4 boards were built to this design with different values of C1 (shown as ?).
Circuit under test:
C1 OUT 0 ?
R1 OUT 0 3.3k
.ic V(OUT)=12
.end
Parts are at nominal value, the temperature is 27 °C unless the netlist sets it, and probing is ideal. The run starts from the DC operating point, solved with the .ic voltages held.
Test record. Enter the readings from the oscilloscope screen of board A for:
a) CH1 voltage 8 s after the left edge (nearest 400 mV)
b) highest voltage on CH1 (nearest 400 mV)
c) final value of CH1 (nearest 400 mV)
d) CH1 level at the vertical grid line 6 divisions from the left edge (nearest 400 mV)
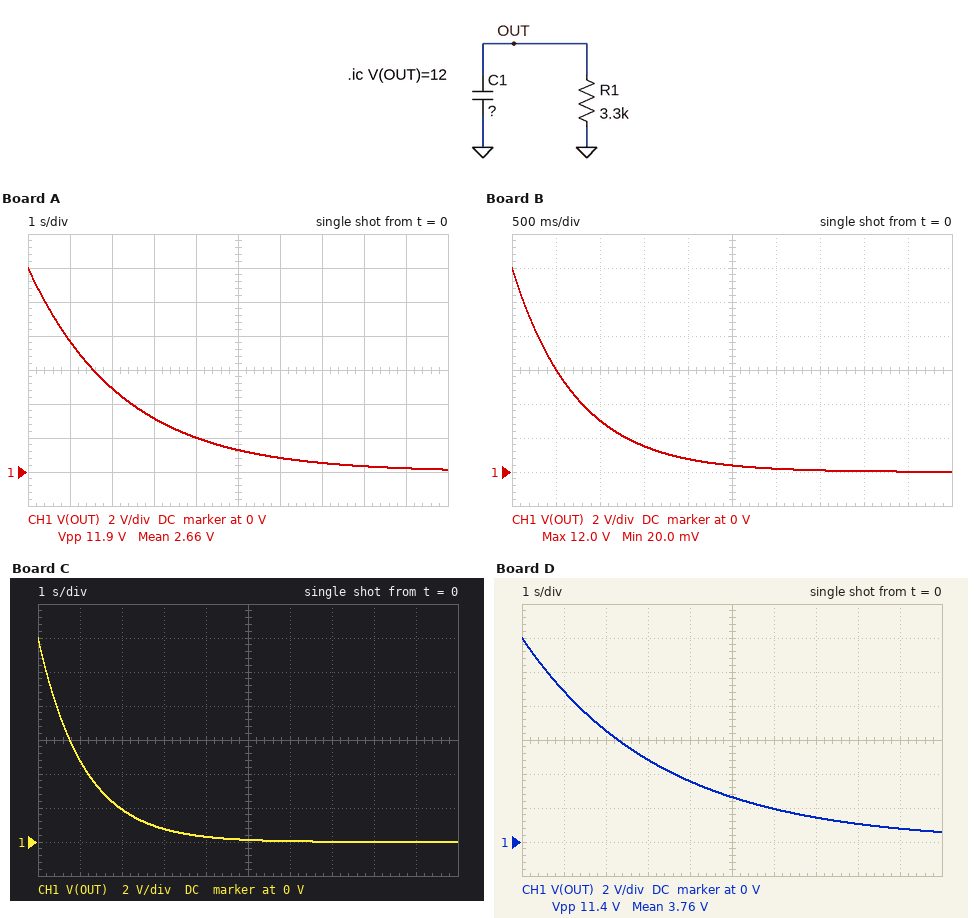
400 mV
12.0 V
0 V
800 mV
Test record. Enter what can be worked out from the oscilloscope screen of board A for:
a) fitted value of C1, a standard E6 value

680 µF
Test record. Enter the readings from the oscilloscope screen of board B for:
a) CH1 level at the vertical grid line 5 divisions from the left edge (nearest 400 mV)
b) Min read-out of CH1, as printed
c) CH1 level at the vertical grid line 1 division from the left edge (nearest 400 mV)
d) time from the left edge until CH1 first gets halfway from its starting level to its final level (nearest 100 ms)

400 mV
20.0 mV
6.0 V
500 ms
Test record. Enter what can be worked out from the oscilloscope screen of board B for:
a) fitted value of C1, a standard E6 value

220 µF
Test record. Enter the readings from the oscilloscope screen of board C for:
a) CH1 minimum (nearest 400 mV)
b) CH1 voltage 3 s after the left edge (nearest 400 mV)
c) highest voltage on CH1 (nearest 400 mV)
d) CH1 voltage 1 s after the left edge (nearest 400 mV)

0 V
800 mV
12.0 V
4.8 V
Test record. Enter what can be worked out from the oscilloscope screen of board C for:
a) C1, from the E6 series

330 µF
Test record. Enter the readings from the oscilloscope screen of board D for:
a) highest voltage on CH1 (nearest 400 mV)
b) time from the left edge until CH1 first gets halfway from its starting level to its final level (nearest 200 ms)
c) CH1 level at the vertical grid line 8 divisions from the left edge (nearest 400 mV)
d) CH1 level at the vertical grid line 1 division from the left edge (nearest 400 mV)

12.0 V
2.2 s
1.2 V
8.8 V
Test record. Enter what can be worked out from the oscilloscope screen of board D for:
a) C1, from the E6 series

1 mF
